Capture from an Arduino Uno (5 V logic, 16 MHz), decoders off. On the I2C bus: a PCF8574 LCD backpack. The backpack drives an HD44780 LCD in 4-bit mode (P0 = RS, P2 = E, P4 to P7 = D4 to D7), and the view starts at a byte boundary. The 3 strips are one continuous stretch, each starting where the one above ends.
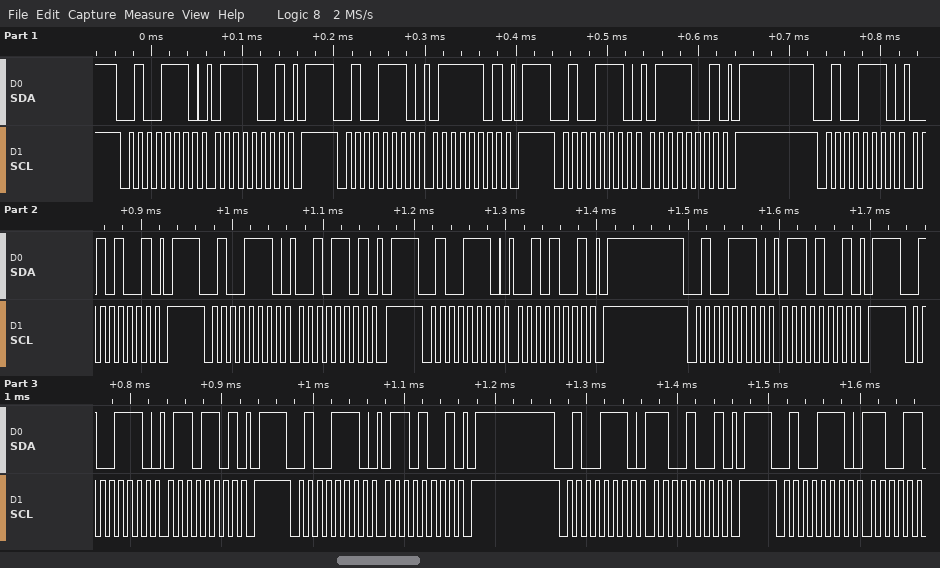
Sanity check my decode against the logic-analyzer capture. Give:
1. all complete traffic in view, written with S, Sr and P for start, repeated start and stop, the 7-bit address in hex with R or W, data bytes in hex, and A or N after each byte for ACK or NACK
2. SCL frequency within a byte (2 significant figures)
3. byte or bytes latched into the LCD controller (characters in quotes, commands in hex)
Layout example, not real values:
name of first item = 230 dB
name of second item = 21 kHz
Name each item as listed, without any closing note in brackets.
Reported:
all complete traffic in view, written with S, Sr and P for start, repeated start and stop, the 7-bit address in hex with R or W, data bytes in hex, and A or N after each byte for ACK or NACK = S 27W A 79 A P S 27W A 7D A P S 27W A 79 A P S 27W A 29 A P S 27W A 2D A P S 27W A 29 A P S 27W A 69 A P S 27W A 6D A P S 27W A 69 A P S 27W A C9 A P S 27W A
SCL frequency within a byte = 100 kHz
byte or bytes latched into the LCD controller = 'r'
